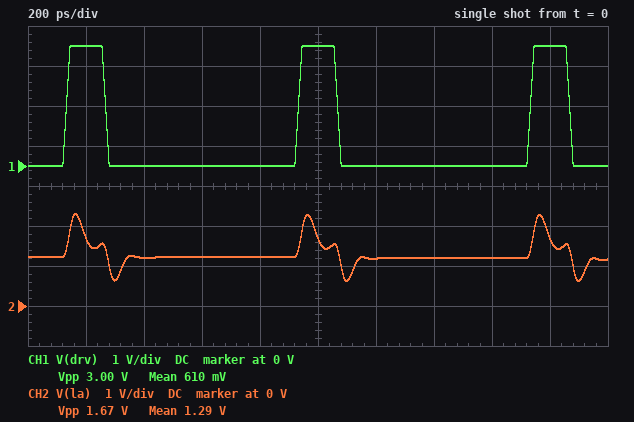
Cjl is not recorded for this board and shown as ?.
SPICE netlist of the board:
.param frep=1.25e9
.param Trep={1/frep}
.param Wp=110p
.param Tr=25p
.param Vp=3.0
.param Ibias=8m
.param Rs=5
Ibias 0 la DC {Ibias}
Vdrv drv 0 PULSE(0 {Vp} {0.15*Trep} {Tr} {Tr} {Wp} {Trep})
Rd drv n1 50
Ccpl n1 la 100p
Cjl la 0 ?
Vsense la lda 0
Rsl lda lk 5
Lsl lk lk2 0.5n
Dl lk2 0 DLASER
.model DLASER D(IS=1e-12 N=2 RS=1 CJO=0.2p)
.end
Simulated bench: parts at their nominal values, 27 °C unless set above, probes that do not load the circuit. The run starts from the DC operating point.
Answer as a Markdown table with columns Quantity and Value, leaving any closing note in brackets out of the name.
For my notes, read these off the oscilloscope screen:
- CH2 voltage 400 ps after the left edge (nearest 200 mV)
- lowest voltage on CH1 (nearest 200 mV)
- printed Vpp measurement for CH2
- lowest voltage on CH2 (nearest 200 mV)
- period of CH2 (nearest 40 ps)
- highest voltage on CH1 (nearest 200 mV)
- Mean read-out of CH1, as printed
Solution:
| Quantity | Value |
|---|---|
| CH2 voltage 400 ps after the left edge | 1.2 V |
| lowest voltage on CH1 | 0 V |
| printed Vpp measurement for CH2 | 1.67 V |
| lowest voltage on CH2 | 600 mV |
| period of CH2 | 800 ps |
| highest voltage on CH1 | 3.0 V |
| Mean read-out of CH1, as printed | 610 mV |
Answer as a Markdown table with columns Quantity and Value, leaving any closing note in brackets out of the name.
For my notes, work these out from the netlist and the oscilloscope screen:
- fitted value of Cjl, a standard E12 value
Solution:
| Quantity | Value |
|---|---|
| fitted value of Cjl, a standard E12 value | 820 fF |
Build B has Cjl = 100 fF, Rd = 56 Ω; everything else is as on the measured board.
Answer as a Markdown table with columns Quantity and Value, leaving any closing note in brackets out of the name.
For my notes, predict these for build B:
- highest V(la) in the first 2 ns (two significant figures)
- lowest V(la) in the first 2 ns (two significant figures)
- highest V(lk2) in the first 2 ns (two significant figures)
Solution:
| Quantity | Value |
|---|---|
| highest V(la) in the first 2 ns | 2.5 V |
| lowest V(la) in the first 2 ns | 350 mV |
| highest V(lk2) in the first 2 ns | 1.3 V |
